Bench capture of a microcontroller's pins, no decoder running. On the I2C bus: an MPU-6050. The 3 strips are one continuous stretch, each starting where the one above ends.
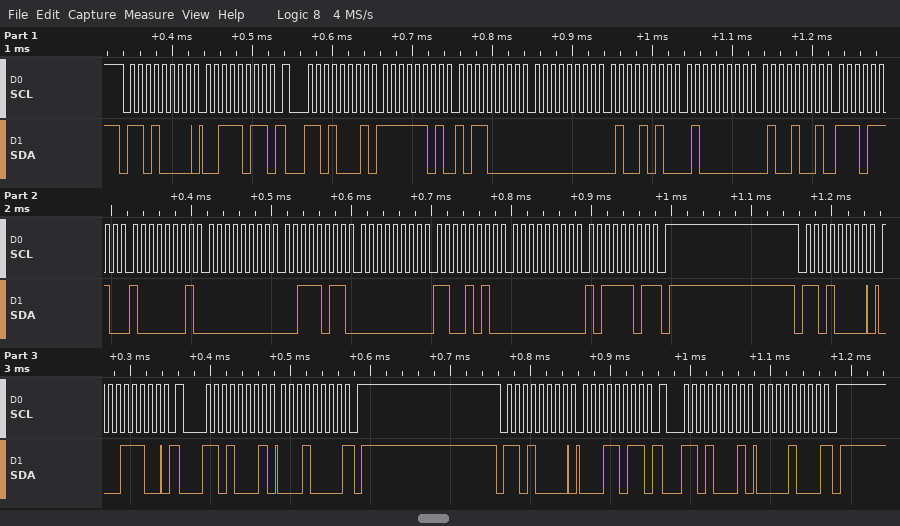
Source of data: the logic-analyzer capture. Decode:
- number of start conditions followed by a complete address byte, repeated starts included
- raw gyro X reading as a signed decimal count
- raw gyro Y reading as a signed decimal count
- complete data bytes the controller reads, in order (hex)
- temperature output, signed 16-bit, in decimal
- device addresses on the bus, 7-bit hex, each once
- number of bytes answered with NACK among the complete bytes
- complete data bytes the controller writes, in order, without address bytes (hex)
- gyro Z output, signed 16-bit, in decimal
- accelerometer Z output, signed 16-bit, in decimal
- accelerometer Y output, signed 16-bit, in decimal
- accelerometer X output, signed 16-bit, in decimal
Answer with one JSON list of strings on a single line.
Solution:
["6", "59", "202", "FD B0 00 4A 40 49 EE 81 00 3B 00 CA 00 BD 10 08", "-4479", "0x68", "3", "3B 1C 1B", "189", "16457", "74", "-592"]
